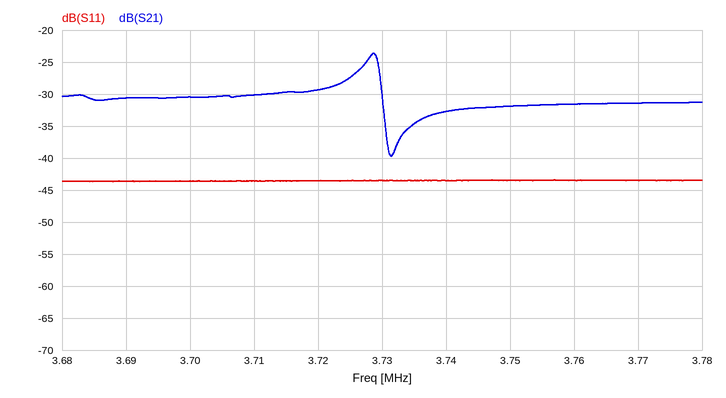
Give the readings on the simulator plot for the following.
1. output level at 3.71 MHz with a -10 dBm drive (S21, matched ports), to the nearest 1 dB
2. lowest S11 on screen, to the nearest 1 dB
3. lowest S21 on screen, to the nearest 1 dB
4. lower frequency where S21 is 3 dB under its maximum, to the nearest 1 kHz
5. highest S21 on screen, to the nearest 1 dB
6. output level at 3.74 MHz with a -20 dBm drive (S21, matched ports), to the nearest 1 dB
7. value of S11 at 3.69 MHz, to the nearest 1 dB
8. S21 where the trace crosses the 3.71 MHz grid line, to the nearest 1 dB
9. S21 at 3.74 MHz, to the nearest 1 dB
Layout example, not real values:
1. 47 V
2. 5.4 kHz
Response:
1. -40 dBm
2. -44 dB
3. -40 dB
4. 3.726 MHz
5. -24 dB
6. -53 dBm
7. -44 dB
8. -30 dB
9. -33 dB
